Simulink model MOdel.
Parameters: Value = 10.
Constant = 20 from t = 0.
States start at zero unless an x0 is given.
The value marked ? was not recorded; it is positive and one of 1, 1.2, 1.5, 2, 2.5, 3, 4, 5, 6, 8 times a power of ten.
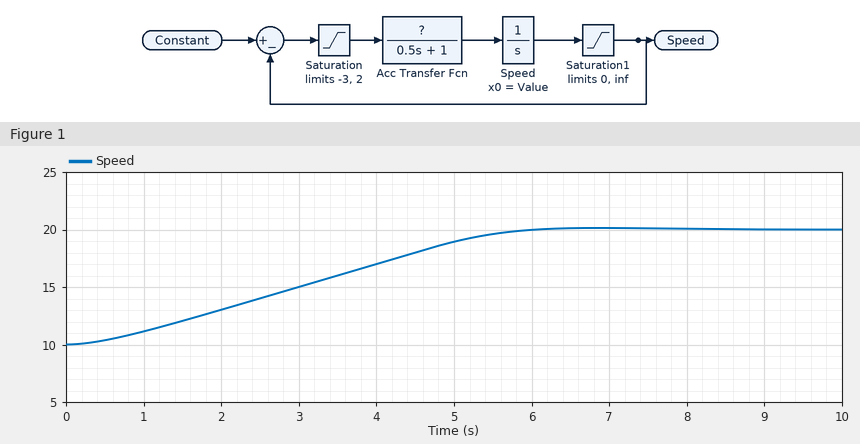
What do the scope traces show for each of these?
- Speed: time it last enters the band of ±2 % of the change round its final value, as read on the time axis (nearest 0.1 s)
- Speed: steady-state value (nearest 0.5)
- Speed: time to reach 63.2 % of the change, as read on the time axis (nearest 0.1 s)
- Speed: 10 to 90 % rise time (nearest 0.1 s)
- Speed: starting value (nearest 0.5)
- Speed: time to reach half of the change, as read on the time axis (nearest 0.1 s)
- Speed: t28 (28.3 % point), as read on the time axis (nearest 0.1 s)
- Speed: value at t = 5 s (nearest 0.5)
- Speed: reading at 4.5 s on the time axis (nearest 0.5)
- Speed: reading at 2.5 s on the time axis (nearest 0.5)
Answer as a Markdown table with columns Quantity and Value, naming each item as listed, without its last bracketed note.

| Quantity | Value |
|---|---|
| Speed: time it last enters the band of ±2 % of the change round its final value, as read on the time axis | 5.7 s |
| Speed: steady-state value | 20.0 |
| Speed: time to reach 63.2 % of the change, as read on the time axis | 3.7 s |
| Speed: 10 to 90 % rise time | 4.1 s |
| Speed: starting value | 10.0 |
| Speed: time to reach half of the change, as read on the time axis | 3.0 s |
| Speed: t28 (28.3 % point), as read on the time axis | 1.9 s |
| Speed: value at t = 5 s | 19.0 |
| Speed: reading at 4.5 s on the time axis | 18.0 |
| Speed: reading at 2.5 s on the time axis | 14.0 |
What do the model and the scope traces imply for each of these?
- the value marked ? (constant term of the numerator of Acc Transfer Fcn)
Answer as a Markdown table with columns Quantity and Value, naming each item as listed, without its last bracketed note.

| Quantity | Value |
|---|---|
| the value marked ? | 1 |
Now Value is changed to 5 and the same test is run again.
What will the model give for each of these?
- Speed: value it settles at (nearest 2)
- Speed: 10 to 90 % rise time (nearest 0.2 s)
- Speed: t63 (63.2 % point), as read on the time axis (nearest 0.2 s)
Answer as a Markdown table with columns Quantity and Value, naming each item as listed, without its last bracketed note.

| Quantity | Value |
|---|---|
| Speed: value it settles at | 20 |
| Speed: 10 to 90 % rise time | 6.0 s |
| Speed: t63 (63.2 % point), as read on the time axis | 5.2 s |
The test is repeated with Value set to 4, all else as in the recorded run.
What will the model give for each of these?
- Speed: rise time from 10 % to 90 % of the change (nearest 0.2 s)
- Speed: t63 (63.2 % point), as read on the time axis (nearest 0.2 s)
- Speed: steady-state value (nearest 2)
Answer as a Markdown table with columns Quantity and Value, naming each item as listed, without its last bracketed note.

| Quantity | Value |
|---|---|
| Speed: rise time from 10 % to 90 % of the change | 6.4 s |
| Speed: t63 (63.2 % point), as read on the time axis | 5.6 s |
| Speed: steady-state value | 20 |
